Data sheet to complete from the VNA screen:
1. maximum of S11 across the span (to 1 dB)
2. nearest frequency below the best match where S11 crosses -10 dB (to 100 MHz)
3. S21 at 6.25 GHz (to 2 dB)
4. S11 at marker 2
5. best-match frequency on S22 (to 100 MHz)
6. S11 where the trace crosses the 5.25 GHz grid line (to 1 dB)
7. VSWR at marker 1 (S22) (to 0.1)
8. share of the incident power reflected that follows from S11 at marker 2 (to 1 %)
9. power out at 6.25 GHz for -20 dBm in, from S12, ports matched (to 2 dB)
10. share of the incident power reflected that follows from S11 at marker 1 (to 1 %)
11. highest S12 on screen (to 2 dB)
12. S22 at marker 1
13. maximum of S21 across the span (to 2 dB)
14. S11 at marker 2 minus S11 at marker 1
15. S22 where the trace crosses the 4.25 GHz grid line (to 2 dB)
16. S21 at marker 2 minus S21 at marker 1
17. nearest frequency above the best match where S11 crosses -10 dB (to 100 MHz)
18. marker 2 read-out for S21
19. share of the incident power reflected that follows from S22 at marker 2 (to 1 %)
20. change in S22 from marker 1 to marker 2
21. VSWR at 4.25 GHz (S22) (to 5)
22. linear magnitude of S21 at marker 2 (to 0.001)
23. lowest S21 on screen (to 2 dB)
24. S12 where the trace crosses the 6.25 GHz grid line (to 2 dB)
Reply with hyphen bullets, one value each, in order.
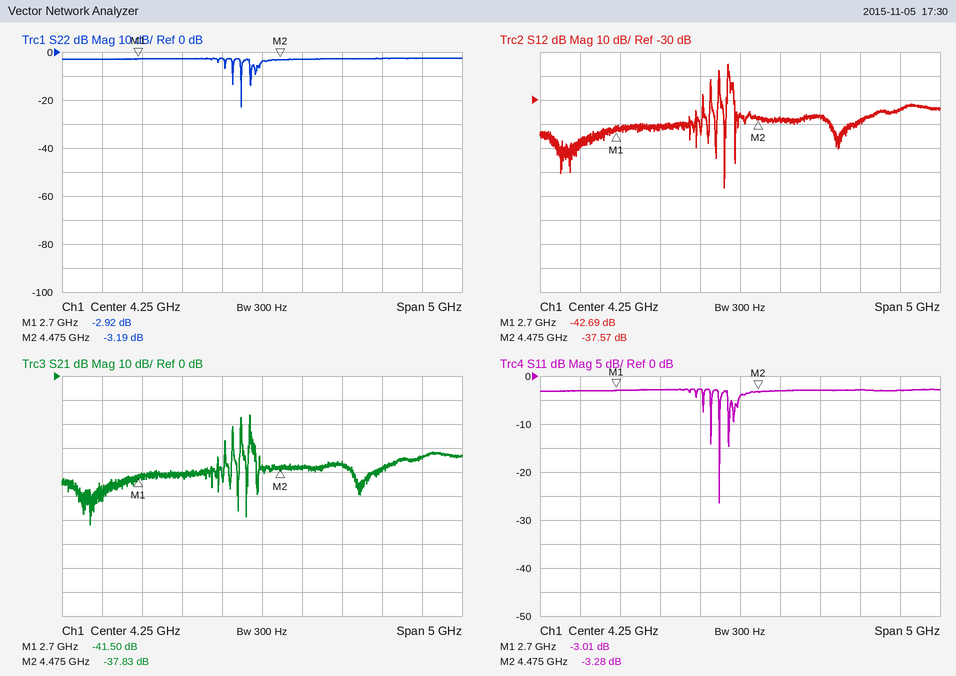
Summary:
- -3 dB
- 4.0 GHz
- -34 dB
- -3.28 dB
- 4.0 GHz
- -3 dB
- 6.0
- 47 %
- -54 dBm
- 50 %
- -16 dB
- -2.92 dB
- -16 dB
- -0.27 dB
- -4 dB
- 3.67 dB
- 4.0 GHz
- -37.83 dB
- 48 %
- -0.27 dB
- 5
- 0.013
- -62 dB
- -34 dB
